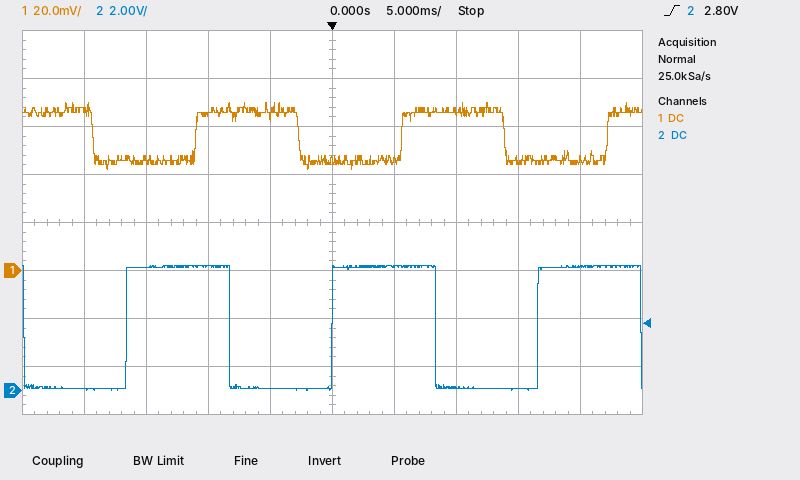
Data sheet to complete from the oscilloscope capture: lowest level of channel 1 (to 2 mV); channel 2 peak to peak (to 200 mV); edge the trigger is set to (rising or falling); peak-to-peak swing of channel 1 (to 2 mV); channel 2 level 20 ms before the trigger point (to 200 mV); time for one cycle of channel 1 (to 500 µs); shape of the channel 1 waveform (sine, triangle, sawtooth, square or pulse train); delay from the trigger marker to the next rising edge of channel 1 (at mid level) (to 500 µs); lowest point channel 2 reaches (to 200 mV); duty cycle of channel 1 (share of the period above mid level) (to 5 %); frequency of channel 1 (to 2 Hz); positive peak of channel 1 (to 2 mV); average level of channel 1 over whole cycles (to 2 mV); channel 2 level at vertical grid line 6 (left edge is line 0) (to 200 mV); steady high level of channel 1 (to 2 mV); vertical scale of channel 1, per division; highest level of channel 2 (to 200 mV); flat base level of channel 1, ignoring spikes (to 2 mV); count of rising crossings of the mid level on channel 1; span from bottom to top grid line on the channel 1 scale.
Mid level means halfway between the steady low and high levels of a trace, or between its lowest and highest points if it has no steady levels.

42 mV
5.2 V
rising
28 mV
0.0 V
16.5 ms
square
5.5 ms
0.0 V
50 %
60 Hz
70 mV
56 mV
5.2 V
66 mV
20 mV
5.2 V
46 mV
3
160 mV
